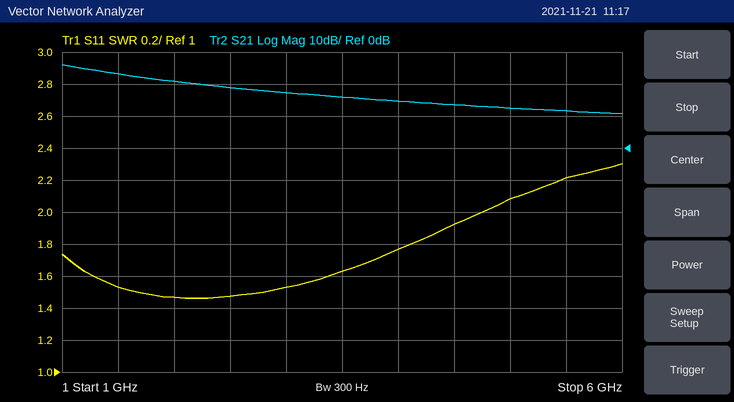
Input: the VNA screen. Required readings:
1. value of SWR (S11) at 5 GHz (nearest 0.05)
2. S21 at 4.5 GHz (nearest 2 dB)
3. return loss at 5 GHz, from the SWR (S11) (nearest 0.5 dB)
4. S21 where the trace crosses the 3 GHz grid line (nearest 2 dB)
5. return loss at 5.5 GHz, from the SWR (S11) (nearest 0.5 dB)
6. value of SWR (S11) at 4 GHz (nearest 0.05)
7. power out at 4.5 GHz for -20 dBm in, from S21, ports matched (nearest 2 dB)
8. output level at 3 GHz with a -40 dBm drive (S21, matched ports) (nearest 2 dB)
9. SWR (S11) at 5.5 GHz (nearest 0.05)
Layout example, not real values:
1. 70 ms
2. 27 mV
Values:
1. 2.10
2. 14 dB
3. 9.0 dB
4. 18 dB
5. 8.5 dB
6. 1.75
7. -6 dBm
8. -22 dBm
9. 2.20
